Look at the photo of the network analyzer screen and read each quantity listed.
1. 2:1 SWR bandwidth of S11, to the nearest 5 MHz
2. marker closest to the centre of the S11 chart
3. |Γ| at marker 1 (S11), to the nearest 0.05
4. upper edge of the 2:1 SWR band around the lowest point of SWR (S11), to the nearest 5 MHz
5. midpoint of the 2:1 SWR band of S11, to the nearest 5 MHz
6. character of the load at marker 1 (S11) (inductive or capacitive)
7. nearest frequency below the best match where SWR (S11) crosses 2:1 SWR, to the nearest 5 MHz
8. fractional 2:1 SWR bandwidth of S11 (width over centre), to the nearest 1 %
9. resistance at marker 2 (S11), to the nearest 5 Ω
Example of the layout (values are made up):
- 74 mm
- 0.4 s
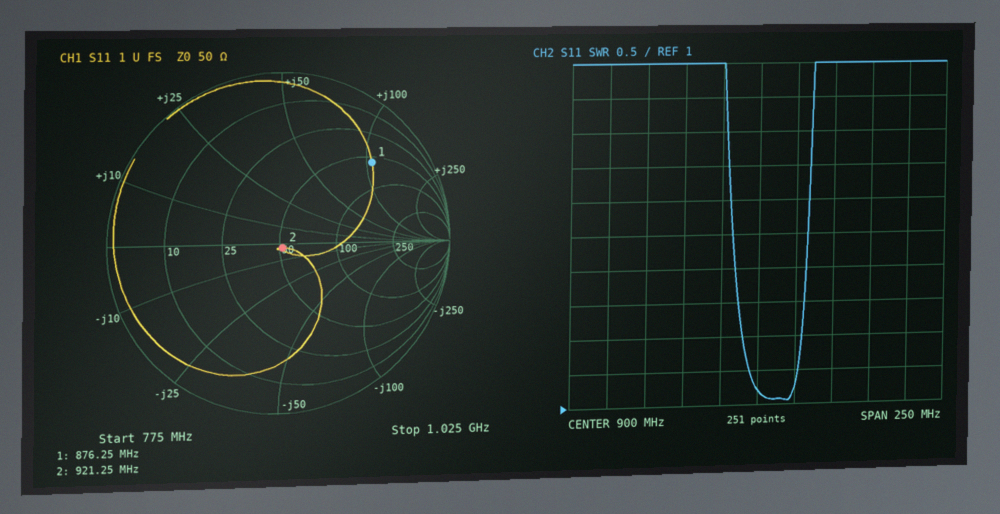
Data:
- 40 MHz
- marker 2
- 0.70
- 930 MHz
- 910 MHz
- inductive
- 890 MHz
- 4 %
- 50 Ω
